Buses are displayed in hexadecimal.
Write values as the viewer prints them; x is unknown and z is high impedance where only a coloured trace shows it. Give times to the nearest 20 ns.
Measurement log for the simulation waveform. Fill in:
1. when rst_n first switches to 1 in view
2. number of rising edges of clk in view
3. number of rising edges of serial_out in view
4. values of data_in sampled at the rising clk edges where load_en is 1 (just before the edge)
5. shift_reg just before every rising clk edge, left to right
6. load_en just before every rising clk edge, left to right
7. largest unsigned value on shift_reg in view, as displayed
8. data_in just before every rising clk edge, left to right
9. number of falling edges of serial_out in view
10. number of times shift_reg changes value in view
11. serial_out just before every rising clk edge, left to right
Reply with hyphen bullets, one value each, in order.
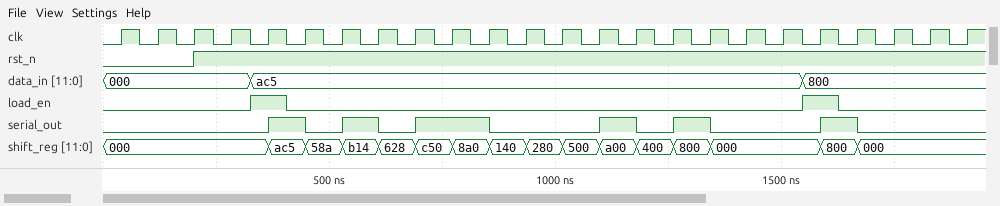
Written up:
- 200 ns
- 24
- 6
- ac5, 800
- 000, 000, 000, 000, 000, ac5, 58a, b14, 628, c50, 8a0, 140, 280, 500, a00, 400, 800, 000, 000, 000, 800, 000, 000, 000
- 0 0 0 0 1 0 0 0 0 0 0 0 0 0 0 0 0 0 0 1 0 0 0 0
- c50
- 000, 000, 000, 000, ac5, ac5, ac5, ac5, ac5, ac5, ac5, ac5, ac5, ac5, ac5, ac5, ac5, ac5, ac5, 800, 800, 800, 800, 800
- 6
- 15
- 0 0 0 0 0 1 0 1 0 1 1 0 0 0 1 0 1 0 0 0 1 0 0 0
